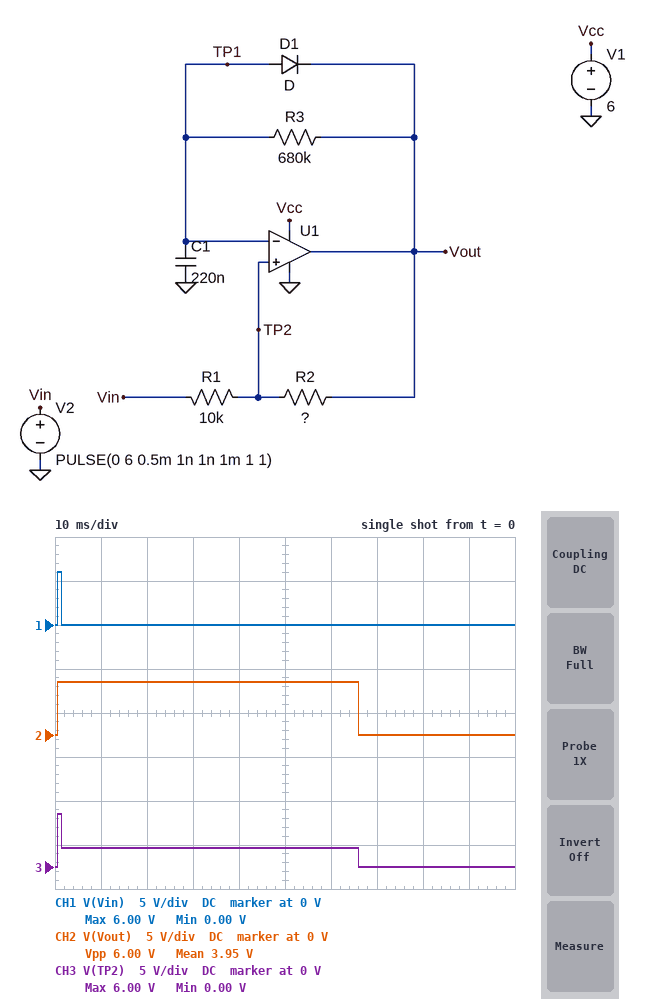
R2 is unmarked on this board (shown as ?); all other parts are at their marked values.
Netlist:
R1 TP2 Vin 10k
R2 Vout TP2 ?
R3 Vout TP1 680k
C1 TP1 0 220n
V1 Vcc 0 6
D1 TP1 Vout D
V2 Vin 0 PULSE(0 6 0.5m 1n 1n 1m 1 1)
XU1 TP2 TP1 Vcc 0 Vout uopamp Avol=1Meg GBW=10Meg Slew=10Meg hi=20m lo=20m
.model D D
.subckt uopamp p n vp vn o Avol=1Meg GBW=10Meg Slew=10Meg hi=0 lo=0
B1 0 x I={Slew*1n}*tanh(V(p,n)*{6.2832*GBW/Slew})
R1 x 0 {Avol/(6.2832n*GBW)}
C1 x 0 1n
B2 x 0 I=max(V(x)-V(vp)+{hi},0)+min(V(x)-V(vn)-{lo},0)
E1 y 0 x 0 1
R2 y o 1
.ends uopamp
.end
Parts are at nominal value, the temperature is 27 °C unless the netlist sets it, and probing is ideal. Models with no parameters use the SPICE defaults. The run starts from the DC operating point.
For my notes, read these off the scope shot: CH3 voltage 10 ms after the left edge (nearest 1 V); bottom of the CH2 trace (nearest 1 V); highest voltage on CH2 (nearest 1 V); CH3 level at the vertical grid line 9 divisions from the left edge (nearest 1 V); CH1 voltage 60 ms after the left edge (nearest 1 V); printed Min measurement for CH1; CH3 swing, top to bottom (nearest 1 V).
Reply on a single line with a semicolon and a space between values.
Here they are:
2 V; 0 V; 6 V; 0 V; 0 V; 0.00 V; 6 V
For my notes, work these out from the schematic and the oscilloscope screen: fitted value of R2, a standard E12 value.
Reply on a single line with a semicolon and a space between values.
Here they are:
18 kΩ
